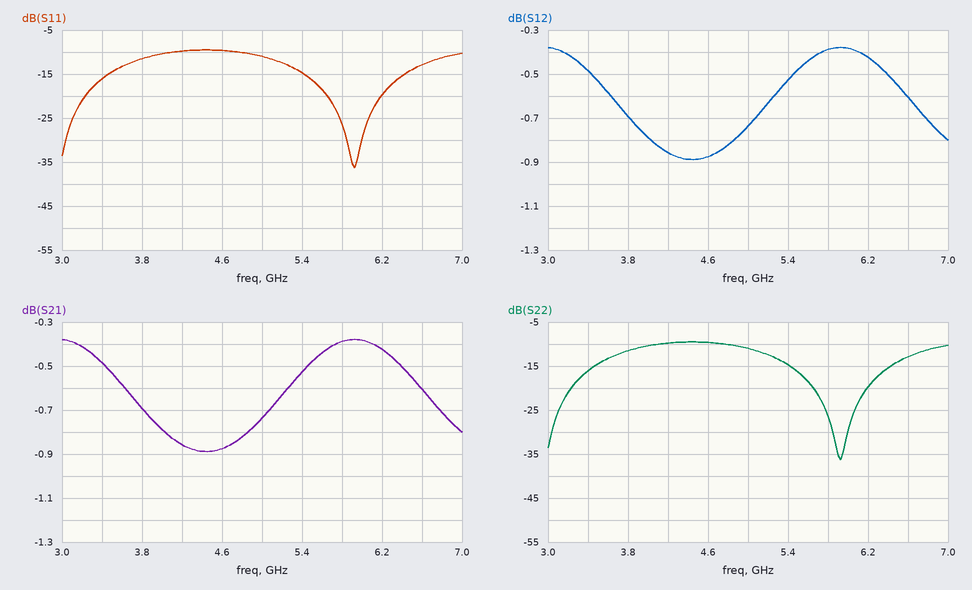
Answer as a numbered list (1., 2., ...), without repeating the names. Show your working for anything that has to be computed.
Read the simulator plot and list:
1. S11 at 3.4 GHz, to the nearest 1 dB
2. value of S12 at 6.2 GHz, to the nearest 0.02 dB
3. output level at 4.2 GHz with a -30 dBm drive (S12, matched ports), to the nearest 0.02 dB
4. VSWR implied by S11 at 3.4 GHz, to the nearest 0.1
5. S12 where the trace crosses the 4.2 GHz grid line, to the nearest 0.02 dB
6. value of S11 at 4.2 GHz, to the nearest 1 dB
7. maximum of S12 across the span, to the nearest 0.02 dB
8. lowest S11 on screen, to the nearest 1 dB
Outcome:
1. -16 dB
2. -0.42 dB
3. -30 dBm + (-0.86 dB) = -30.86 dBm
4. |Γ| = 10^(-16/20) = 0.1585; VSWR = (1 + 0.1585)/(1 − 0.1585) ≈ 1.4
5. -0.86 dB
6. -10 dB
7. -0.38 dB
8. -36 dB
